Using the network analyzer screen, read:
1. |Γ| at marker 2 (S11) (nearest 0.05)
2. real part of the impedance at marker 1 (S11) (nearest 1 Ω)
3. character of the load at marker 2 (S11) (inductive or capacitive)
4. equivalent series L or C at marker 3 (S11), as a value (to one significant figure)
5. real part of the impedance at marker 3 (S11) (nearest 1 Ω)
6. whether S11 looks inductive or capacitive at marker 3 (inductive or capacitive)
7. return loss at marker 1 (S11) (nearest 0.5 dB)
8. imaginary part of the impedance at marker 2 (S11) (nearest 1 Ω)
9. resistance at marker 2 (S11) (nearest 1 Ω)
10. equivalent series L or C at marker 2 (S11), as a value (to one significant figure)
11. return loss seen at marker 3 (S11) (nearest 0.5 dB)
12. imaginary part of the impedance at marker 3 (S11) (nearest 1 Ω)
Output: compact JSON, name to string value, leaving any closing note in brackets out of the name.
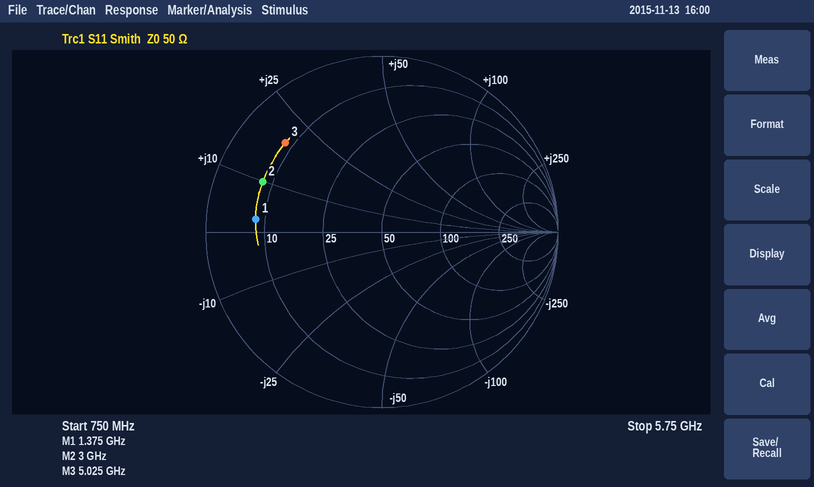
{"|Γ| at marker 2 (S11)": "0.75", "real part of the impedance at marker 1 (S11)": "8 Ω", "character of the load at marker 2 (S11)": "inductive", "equivalent series L or C at marker 3 (S11), as a value": "600 pH", "real part of the impedance at marker 3 (S11)": "8 Ω", "whether S11 looks inductive or capacitive at marker 3": "inductive", "return loss at marker 1 (S11)": "3.0 dB", "imaginary part of the impedance at marker 2 (S11)": "+10 Ω", "resistance at marker 2 (S11)": "8 Ω", "equivalent series L or C at marker 2 (S11), as a value": "500 pH", "return loss seen at marker 3 (S11)": "2.5 dB", "imaginary part of the impedance at marker 3 (S11)": "+19 Ω"}
